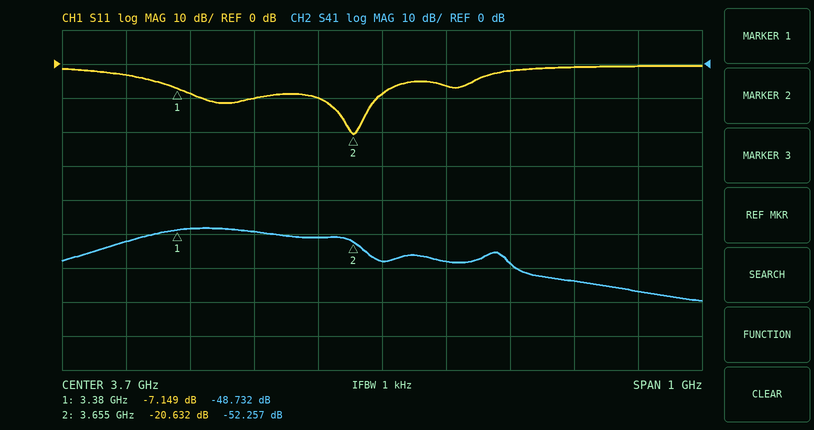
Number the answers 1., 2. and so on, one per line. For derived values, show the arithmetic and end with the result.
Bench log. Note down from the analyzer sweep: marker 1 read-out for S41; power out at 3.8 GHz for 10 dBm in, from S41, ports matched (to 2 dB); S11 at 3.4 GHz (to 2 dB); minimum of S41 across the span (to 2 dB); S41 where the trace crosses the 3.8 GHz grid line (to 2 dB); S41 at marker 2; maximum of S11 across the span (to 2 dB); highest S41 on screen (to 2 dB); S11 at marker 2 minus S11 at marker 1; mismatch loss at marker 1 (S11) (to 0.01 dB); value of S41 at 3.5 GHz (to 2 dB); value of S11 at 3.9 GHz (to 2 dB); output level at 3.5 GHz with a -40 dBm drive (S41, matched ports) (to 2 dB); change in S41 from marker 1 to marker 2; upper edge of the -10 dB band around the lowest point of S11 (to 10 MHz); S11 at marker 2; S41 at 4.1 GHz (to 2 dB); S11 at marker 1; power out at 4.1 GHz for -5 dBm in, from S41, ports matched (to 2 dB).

1. -48.732 dB
2. 10 dBm + (-58 dB) = -48 dBm
3. -8 dB
4. -70 dB
5. -58 dB
6. -52.257 dB
7. 0 dB
8. -48 dB
9. -20.632 − (-7.149) = -13.483 dB
10. −10 log10(1 − 10^(-7.149/10)) ≈ 0.93 dB
11. -50 dB
12. -2 dB
13. -40 dBm + (-50 dB) = -90 dBm
14. -52.257 − (-48.732) = -3.525 dB
15. 3.69 GHz
16. -20.632 dB
17. -66 dB
18. -7.149 dB
19. -5 dBm + (-66 dB) = -72 dBm
